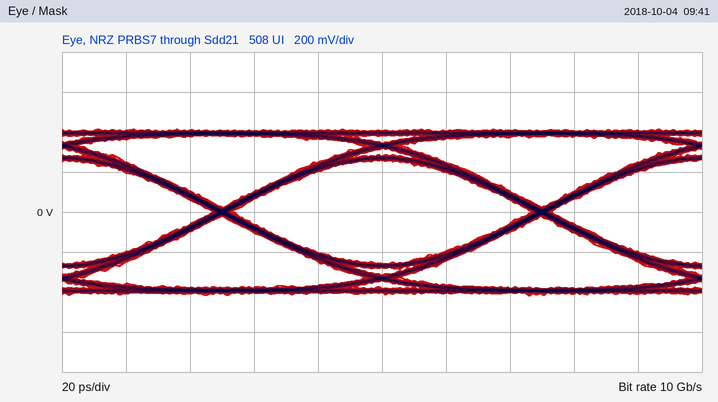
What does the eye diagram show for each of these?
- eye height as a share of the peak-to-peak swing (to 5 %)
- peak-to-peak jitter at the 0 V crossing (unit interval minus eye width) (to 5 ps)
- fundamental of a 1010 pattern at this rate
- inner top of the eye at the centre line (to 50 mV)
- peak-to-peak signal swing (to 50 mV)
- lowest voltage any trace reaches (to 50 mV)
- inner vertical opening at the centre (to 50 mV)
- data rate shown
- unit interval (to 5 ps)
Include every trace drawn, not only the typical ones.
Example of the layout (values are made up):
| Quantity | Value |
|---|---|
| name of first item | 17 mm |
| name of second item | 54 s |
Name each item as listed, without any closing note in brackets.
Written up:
| Quantity | Value |
|---|---|
| eye height as a share of the peak-to-peak swing | 60 % |
| peak-to-peak jitter at the 0 V crossing (unit interval minus eye width) | 5 ps |
| fundamental of a 1010 pattern at this rate | 5 GHz |
| inner top of the eye at the centre line | 250 mV |
| peak-to-peak signal swing | 850 mV |
| lowest voltage any trace reaches | -400 mV |
| inner vertical opening at the centre | 500 mV |
| data rate shown | 10 Gb/s |
| unit interval | 100 ps |
